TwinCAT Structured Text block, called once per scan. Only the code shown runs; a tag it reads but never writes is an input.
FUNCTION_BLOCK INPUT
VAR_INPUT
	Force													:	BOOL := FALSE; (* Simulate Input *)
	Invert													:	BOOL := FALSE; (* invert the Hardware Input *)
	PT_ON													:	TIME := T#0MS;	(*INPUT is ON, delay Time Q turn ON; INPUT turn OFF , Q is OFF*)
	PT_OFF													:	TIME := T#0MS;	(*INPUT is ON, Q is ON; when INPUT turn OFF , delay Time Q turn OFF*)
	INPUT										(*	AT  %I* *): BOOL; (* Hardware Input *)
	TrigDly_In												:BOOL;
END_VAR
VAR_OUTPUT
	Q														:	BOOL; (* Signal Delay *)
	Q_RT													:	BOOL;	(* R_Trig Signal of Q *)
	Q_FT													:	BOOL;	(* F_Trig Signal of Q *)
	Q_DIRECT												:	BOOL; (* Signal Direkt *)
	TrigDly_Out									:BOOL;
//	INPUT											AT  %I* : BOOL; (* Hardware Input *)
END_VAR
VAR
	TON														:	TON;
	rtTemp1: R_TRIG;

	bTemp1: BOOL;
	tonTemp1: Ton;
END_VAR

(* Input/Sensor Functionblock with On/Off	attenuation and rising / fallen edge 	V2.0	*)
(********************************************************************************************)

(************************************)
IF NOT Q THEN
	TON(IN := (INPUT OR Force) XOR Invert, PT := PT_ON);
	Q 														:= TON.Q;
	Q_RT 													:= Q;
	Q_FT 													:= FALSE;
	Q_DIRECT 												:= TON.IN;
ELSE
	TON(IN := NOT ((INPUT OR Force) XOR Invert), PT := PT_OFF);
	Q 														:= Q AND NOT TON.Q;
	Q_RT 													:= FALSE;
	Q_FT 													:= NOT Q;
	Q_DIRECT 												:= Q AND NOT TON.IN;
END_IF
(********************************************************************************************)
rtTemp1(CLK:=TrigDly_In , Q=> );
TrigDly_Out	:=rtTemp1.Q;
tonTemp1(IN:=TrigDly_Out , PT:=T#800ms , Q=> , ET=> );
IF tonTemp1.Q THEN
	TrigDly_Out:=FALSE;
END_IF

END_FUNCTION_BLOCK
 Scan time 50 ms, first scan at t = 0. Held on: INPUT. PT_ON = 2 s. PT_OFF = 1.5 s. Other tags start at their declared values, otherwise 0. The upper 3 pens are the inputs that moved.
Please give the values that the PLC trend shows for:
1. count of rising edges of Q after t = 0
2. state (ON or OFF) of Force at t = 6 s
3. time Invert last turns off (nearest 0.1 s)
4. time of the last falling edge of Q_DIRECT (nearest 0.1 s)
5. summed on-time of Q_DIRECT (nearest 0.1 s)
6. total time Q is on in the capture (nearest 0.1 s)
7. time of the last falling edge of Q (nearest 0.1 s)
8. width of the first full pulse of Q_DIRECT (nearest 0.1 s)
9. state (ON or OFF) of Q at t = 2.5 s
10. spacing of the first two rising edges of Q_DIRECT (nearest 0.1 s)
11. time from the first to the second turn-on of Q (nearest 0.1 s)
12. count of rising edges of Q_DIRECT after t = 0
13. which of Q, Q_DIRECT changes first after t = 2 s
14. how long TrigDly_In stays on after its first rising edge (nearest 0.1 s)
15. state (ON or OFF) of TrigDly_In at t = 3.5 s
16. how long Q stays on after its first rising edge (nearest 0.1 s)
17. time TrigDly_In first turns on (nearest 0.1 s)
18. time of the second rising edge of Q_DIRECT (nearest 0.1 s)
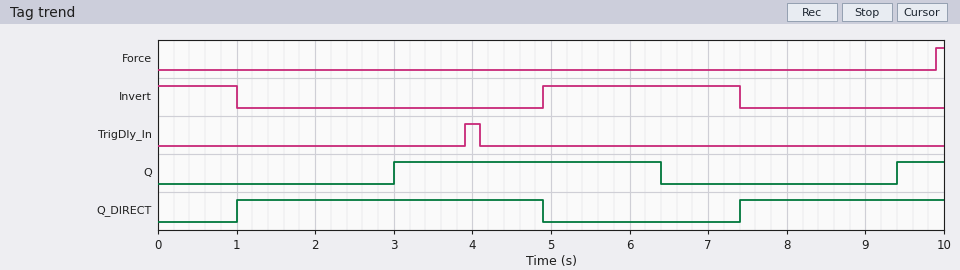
2
OFF
7.4 s
4.9 s
6.5 s
4.0 s
6.4 s
3.9 s
OFF
6.4 s
6.4 s
2
Q
0.2 s
OFF
3.4 s
3.9 s
7.4 s
